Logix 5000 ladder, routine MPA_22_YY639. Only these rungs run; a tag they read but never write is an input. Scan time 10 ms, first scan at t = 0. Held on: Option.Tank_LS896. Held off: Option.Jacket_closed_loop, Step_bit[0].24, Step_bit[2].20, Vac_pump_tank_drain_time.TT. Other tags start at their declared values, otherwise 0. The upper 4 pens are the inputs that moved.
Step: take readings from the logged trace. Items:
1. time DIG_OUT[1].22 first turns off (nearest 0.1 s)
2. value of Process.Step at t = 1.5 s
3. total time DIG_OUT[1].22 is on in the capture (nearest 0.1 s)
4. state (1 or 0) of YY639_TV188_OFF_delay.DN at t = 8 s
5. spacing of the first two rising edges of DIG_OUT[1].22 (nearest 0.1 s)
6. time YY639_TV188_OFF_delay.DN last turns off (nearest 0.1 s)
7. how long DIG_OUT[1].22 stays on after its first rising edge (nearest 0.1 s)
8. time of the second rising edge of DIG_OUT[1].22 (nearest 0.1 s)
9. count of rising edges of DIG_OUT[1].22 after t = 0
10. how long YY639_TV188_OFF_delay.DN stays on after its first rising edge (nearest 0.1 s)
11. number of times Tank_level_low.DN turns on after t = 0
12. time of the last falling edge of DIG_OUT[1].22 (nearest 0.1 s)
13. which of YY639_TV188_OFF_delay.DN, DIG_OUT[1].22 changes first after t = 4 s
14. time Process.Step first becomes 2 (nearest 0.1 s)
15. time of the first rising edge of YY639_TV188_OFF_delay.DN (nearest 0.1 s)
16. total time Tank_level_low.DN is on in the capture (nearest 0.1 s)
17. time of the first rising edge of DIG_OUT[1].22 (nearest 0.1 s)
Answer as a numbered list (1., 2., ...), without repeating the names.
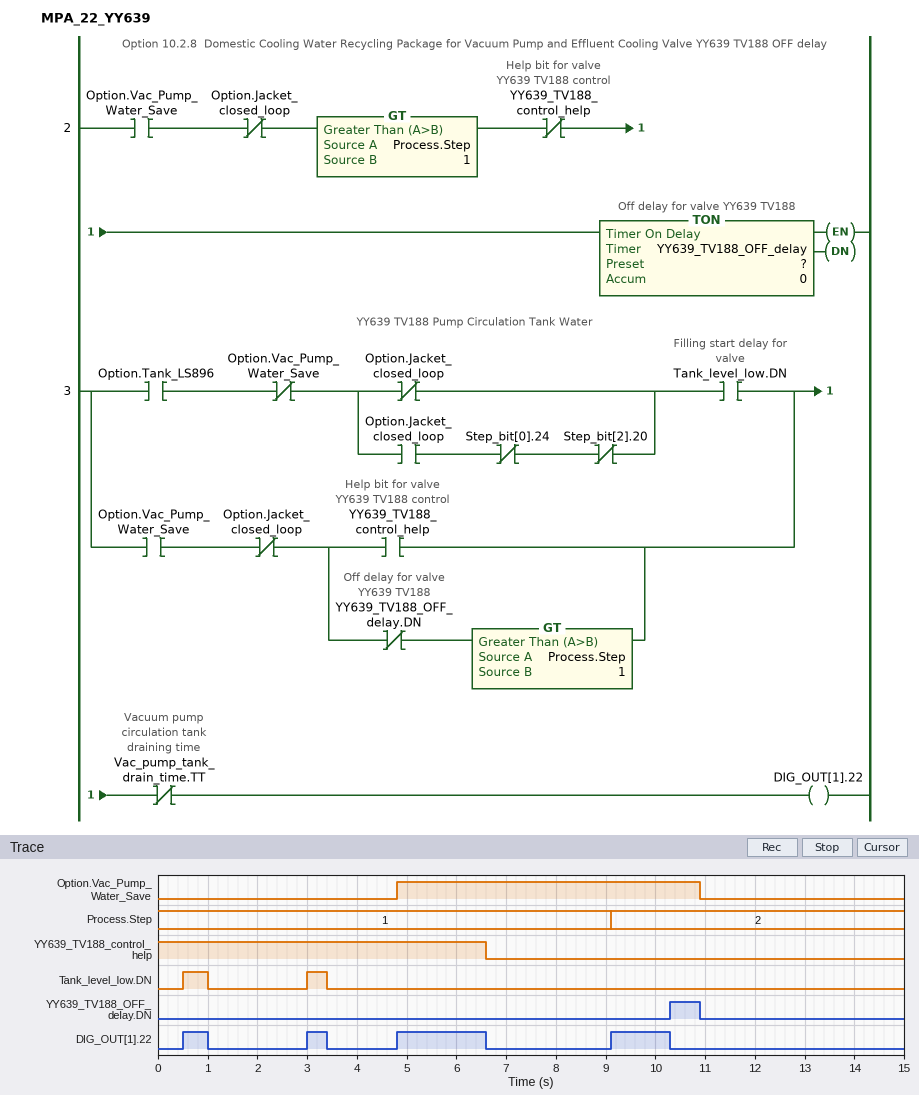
1. 1.0 s
2. 1
3. 3.9 s
4. 0
5. 2.5 s
6. 10.9 s
7. 0.5 s
8. 3.0 s
9. 4
10. 0.6 s
11. 2
12. 10.3 s
13. DIG_OUT[1].22
14. 9.1 s
15. 10.3 s
16. 0.9 s
17. 0.5 s
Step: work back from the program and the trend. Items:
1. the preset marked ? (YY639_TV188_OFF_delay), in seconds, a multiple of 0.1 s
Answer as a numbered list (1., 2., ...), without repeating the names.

1. 1.2 s
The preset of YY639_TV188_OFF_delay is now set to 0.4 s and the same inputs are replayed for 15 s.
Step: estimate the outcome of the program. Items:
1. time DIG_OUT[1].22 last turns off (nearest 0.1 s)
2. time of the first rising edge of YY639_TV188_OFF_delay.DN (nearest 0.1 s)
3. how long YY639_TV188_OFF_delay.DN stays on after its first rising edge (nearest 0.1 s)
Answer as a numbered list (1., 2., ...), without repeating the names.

1. 9.5 s
2. 9.5 s
3. 1.4 s
